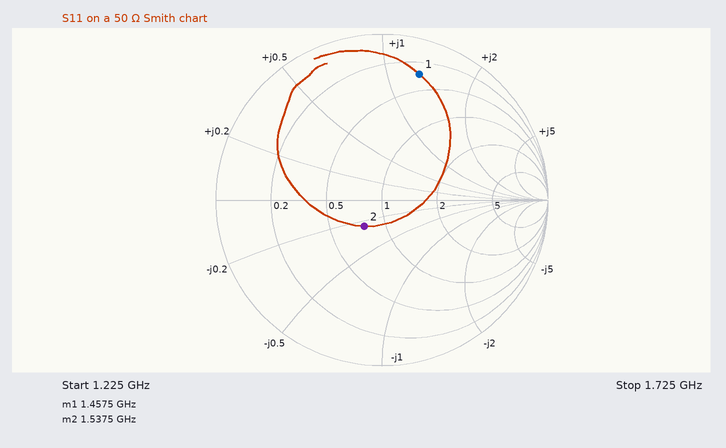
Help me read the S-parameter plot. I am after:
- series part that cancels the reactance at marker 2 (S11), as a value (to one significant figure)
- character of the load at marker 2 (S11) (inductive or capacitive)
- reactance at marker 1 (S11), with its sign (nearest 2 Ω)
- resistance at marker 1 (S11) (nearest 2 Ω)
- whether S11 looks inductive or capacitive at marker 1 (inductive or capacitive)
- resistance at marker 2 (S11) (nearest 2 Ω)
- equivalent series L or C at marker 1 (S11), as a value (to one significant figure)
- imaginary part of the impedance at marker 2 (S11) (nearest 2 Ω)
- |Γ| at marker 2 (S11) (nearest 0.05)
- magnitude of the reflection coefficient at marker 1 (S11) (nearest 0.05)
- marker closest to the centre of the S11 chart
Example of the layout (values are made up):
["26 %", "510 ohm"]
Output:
["1 nH", "capacitive", "+64 Ω", "16 Ω", "inductive", "38 Ω", "7 nH", "-12 Ω", "0.20", "0.80", "marker 2"]
